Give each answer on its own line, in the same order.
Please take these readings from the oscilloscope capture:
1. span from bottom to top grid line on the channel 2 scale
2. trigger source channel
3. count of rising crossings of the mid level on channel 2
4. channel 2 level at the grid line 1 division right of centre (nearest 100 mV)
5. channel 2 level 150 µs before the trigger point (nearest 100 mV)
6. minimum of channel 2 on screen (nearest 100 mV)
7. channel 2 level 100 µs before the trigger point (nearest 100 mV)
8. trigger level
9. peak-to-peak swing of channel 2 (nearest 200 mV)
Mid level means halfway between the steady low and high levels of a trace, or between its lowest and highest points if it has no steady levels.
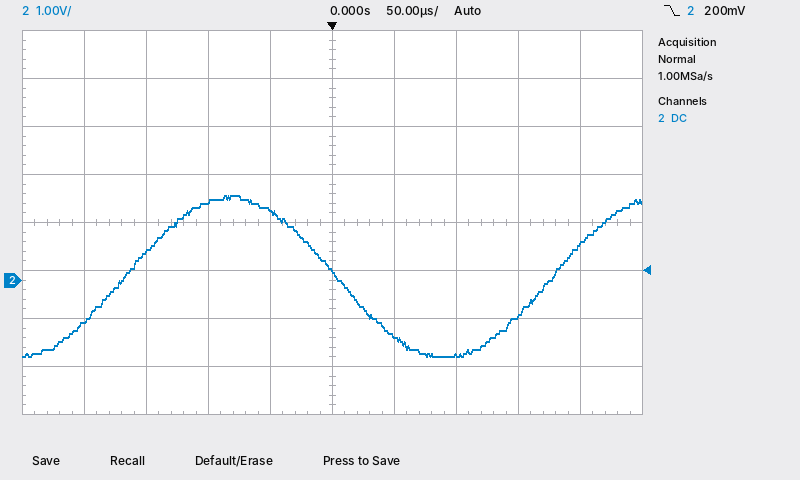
8 V
channel 2
2
-1.2 V
600 mV
-1.6 V
1.6 V
200 mV
3.4 V
